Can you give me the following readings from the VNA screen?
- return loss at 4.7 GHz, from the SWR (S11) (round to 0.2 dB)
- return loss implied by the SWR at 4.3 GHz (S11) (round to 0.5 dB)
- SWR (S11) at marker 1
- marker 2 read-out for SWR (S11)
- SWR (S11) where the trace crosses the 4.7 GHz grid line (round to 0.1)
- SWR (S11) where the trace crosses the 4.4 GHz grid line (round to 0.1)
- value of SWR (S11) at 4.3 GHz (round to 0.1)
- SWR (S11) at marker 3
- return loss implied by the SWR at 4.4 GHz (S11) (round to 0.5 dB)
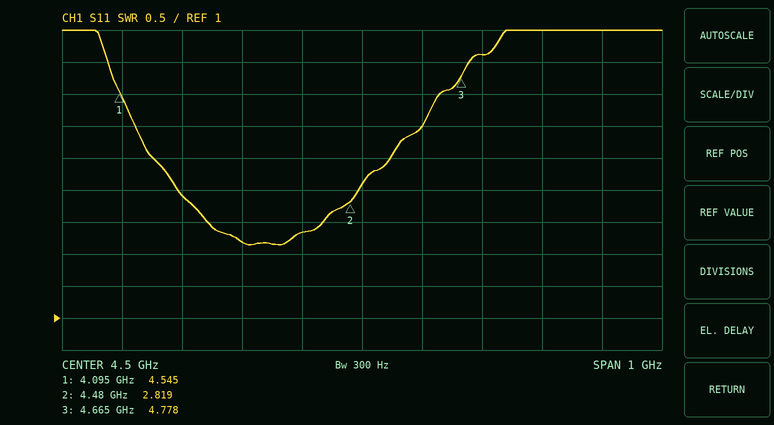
3.4 dB
8.5 dB
4.545
2.819
5.1
2.3
2.2
4.778
8.0 dB
